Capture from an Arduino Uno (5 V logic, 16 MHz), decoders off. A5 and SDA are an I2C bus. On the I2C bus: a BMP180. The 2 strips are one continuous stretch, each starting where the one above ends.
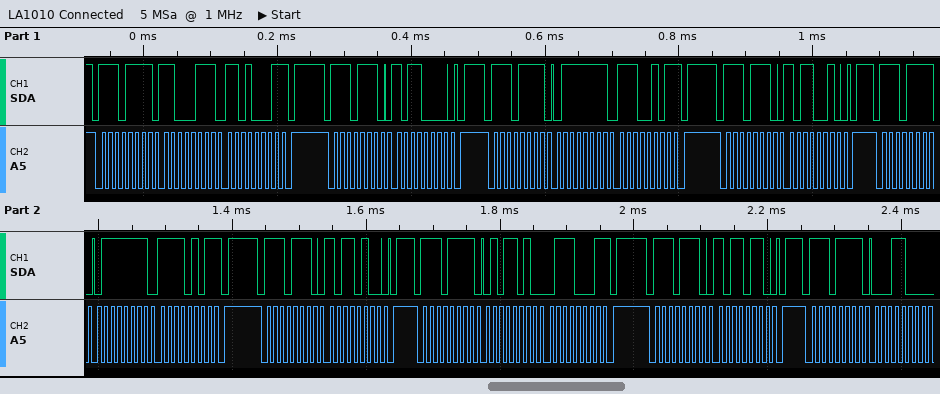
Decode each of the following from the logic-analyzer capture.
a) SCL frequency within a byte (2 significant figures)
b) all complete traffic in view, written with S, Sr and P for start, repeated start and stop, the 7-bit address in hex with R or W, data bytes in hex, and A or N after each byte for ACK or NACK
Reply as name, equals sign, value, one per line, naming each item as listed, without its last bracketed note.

SCL frequency within a byte = 100 kHz
all complete traffic in view, written with S, Sr and P for start, repeated start and stop, the 7-bit address in hex with R or W, data bytes in hex, and A or N after each byte for ACK or NACK = S 77R A C7 A D1 N P S 77W A B0 A P S 77R A 7F A E5 N P S 77W A B2 A P S 77R A 7F A F5 N P S 77W A B4 A P S 77R A 5A A 71 N P S 77W A B6 A P S 77R A 18 A
